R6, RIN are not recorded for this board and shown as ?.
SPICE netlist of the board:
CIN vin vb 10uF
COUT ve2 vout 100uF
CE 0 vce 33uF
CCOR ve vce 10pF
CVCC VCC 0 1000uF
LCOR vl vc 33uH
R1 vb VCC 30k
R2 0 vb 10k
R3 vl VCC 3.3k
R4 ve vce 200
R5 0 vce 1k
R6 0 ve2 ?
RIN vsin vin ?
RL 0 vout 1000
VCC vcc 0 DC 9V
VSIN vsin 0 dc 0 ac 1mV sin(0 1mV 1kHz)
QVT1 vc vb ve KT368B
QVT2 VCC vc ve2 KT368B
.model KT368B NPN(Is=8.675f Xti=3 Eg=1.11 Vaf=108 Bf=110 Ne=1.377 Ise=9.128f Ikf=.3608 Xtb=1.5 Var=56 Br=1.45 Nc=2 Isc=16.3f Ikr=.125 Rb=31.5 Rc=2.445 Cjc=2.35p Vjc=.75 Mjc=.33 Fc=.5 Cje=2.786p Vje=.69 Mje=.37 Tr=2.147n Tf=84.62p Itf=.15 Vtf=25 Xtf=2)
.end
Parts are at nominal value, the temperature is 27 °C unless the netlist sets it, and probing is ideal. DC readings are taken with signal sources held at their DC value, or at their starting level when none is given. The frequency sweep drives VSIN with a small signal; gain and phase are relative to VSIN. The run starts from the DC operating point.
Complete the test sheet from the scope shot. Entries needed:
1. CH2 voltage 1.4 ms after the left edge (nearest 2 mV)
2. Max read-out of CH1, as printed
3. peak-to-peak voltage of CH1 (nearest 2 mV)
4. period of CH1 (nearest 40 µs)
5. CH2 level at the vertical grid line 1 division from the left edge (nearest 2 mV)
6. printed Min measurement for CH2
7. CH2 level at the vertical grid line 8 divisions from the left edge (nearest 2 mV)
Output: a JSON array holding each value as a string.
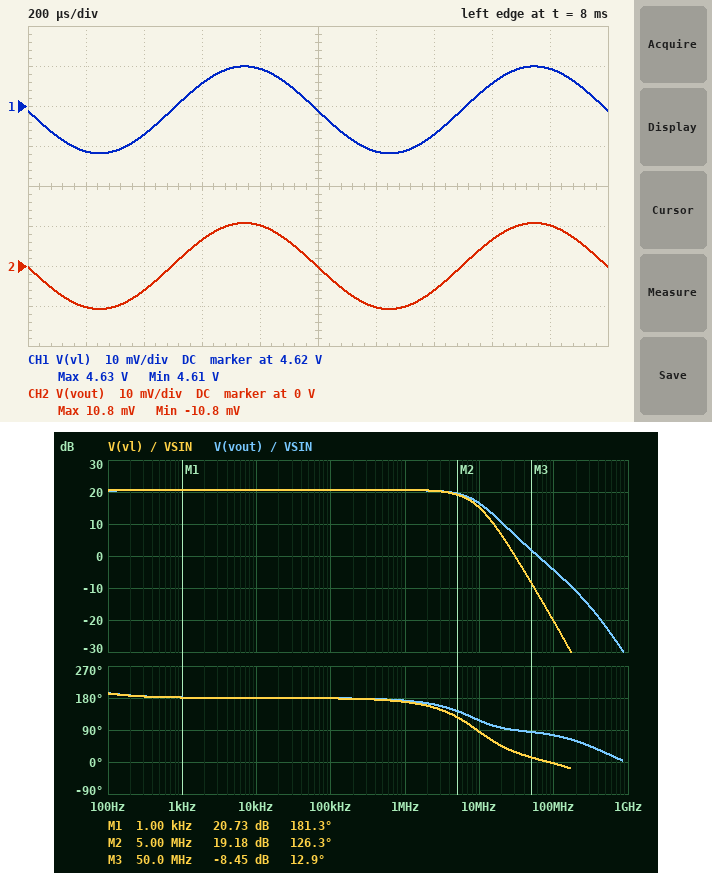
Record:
["-6 mV", "4.63 V", "22 mV", "1.00 ms", "-10 mV", "-10.8 mV", "6 mV"]
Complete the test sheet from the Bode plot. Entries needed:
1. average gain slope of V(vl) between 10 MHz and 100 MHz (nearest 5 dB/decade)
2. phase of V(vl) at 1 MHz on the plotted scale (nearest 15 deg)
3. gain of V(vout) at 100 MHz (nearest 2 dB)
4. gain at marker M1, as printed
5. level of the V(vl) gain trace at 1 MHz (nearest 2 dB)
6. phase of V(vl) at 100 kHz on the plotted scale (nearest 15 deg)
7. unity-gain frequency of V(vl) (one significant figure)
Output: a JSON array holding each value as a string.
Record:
["-35 dB/decade", "165 deg", "-4 dB", "20.73 dB", "20 dB", "180 deg", "30 MHz"]
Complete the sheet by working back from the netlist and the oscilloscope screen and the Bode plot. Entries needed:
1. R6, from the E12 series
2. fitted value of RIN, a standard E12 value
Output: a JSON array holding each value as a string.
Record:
["390 Ω", "1.2 kΩ"]
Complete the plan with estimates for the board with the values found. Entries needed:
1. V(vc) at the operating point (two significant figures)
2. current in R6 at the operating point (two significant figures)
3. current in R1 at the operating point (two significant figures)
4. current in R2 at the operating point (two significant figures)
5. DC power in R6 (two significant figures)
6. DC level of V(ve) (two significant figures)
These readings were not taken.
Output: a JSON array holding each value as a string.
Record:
["4.6 V", "10 mA", "230 µA", "220 µA", "39 mW", "1.5 V"]
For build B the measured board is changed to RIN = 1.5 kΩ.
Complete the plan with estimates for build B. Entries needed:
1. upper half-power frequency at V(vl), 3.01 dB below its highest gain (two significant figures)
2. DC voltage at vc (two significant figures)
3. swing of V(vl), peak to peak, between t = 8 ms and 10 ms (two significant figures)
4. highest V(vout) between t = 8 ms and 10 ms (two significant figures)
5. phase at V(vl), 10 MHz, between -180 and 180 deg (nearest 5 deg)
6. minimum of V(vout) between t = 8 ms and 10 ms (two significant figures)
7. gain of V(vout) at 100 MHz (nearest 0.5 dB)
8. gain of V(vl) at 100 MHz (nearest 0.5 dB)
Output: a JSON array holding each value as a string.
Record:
["6.0 MHz", "4.6 V", "21 mV", "10 mV", "80 deg", "-10 mV", "-6.0 dB", "-22.0 dB"]
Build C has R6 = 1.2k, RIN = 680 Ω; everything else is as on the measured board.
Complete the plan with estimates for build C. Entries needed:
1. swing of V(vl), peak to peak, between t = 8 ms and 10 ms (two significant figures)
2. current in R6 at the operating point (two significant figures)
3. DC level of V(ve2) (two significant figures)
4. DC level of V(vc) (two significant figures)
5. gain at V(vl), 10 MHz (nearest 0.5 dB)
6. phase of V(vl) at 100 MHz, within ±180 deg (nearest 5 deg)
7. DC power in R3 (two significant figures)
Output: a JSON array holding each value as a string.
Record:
["25 mV", "3.4 mA", "4.1 V", "4.8 V", "19.0 dB", "0 deg", "5.3 mW"]
